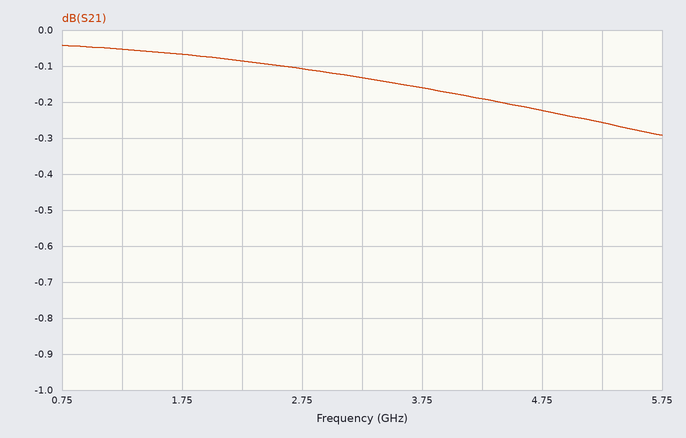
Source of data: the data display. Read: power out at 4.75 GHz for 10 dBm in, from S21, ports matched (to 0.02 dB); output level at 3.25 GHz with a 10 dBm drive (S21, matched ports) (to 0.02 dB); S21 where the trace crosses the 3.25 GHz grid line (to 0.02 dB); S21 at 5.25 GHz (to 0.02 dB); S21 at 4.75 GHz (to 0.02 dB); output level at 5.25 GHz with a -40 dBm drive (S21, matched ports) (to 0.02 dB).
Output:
9.78 dBm
9.86 dBm
-0.14 dB
-0.26 dB
-0.22 dB
-40.26 dBm
